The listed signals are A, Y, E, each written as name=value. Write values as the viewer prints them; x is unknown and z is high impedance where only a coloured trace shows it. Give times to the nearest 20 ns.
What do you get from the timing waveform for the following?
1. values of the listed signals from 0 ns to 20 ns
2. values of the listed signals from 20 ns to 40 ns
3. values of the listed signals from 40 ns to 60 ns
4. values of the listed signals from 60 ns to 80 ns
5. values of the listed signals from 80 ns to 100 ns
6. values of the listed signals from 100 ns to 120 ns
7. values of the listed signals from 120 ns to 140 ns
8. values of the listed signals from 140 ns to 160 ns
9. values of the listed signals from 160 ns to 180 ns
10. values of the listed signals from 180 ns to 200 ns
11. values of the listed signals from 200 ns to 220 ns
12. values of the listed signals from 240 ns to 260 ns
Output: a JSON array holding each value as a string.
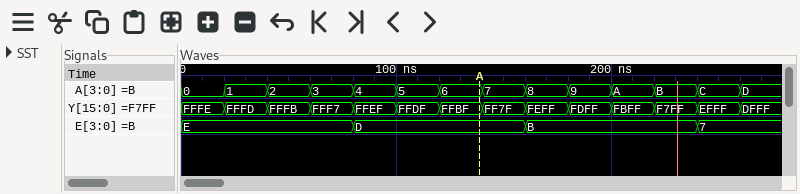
["A=0, Y=FFFE, E=E", "A=1, Y=FFFD, E=E", "A=2, Y=FFFB, E=E", "A=3, Y=FFF7, E=E", "A=4, Y=FFEF, E=D", "A=5, Y=FFDF, E=D", "A=6, Y=FFBF, E=D", "A=7, Y=FF7F, E=D", "A=8, Y=FEFF, E=B", "A=9, Y=FDFF, E=B", "A=A, Y=FBFF, E=B", "A=C, Y=EFFF, E=7"]
